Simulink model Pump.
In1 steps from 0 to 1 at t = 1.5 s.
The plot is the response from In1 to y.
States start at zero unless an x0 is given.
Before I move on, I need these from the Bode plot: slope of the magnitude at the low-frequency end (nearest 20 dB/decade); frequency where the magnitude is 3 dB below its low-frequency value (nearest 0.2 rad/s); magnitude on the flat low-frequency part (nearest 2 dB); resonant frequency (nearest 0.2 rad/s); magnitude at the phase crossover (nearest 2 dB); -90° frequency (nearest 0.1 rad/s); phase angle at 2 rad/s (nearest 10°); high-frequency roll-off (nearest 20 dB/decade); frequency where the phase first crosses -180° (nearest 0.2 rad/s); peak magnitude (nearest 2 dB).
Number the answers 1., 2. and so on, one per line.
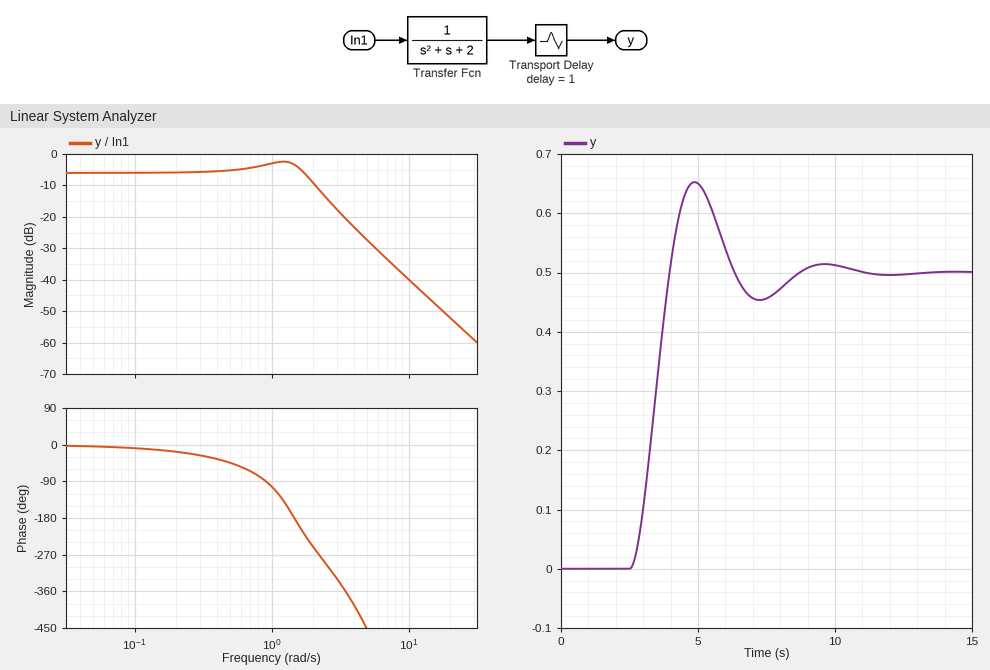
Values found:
1. 0 dB/decade
2. 2.0 rad/s
3. -6 dB
4. 1.2 rad/s
5. -4 dB
6. 0.9 rad/s
7. -250°
8. -40 dB/decade
9. 1.4 rad/s
10. -2 dB
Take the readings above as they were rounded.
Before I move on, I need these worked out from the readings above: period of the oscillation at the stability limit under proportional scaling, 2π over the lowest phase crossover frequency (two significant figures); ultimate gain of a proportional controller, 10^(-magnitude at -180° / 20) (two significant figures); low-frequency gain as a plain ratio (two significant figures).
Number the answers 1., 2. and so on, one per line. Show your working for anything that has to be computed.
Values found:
1. 2π / 1.4 = 4.5 s
2. 10^(4 / 20) = 1.6
3. 10^(-6 / 20) = 0.50
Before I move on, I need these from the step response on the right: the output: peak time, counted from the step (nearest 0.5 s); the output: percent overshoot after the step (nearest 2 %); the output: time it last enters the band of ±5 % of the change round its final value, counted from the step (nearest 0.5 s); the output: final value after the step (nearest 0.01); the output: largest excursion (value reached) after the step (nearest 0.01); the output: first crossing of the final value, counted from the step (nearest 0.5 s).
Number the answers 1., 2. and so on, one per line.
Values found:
1. 3.5 s
2. 30 %
3. 6.5 s
4. 0.50
5. 0.65
6. 2.5 s
